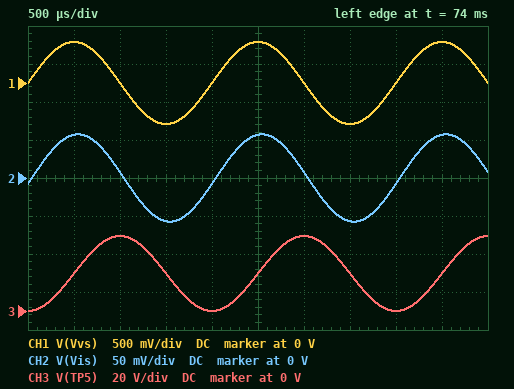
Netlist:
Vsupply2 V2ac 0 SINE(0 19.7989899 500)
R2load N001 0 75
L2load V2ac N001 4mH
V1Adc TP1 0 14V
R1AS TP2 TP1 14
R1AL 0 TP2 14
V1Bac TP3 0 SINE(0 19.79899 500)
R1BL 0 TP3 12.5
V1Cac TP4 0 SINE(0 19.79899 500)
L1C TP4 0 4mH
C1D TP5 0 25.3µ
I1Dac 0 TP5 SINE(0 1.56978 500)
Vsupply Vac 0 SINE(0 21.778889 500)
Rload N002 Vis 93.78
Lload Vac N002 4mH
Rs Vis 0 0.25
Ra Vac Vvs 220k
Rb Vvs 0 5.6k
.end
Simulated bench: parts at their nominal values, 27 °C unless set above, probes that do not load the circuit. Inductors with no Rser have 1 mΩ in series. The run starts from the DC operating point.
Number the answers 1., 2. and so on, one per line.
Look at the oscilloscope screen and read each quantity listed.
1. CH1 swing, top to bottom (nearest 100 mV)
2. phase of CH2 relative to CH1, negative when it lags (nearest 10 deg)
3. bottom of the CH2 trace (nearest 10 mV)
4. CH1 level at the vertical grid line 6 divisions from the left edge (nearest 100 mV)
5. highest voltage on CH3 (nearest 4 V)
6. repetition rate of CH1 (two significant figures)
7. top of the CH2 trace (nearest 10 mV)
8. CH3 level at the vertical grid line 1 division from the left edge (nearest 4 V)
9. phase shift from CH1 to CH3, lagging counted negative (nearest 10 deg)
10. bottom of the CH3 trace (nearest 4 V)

1. 1.1 V
2. -10 deg
3. -60 mV
4. 0 V
5. 40 V
6. 500 Hz
7. 60 mV
8. 20 V
9. -90 deg
10. 0 V
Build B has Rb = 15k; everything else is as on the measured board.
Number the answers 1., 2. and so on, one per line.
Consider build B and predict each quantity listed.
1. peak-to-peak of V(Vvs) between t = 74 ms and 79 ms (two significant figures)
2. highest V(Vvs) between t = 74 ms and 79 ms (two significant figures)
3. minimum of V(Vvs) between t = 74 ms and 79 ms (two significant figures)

1. 2.8 V
2. 1.4 V
3. -1.4 V
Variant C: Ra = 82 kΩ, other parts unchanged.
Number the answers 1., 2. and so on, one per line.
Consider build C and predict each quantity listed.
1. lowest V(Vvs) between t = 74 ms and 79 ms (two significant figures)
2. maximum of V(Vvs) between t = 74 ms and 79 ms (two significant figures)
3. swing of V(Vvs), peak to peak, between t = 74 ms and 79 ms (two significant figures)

1. -1.4 V
2. 1.4 V
3. 2.8 V
